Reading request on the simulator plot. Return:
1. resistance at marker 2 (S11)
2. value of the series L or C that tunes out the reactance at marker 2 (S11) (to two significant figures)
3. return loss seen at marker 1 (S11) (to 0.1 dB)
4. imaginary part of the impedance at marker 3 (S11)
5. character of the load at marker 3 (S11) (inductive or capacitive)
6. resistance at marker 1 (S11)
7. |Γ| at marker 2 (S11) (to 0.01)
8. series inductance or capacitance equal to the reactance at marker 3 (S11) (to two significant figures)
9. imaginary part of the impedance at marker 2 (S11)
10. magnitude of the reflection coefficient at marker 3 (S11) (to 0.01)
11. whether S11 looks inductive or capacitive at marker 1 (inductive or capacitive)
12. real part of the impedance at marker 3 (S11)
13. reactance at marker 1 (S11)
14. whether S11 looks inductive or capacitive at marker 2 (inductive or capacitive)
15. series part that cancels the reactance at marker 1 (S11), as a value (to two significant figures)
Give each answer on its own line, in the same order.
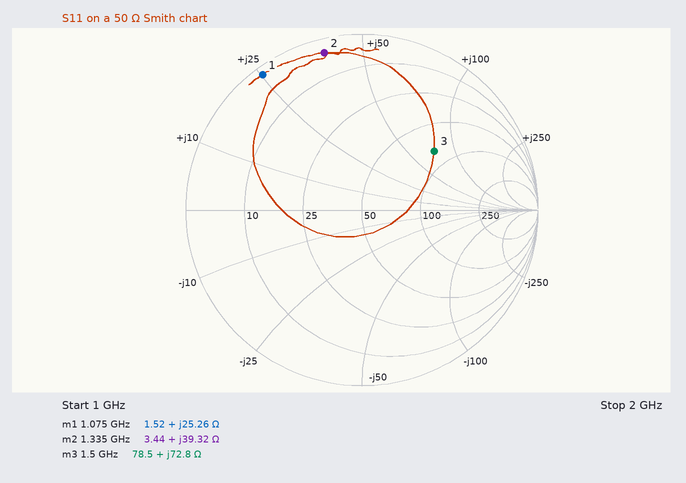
3.44 Ω
3.0 pF
0.4 dB
+72.8 Ω
inductive
1.52 Ω
0.92
7.7 nH
+39.32 Ω
0.53
inductive
78.5 Ω
+25.26 Ω
inductive
5.9 pF
